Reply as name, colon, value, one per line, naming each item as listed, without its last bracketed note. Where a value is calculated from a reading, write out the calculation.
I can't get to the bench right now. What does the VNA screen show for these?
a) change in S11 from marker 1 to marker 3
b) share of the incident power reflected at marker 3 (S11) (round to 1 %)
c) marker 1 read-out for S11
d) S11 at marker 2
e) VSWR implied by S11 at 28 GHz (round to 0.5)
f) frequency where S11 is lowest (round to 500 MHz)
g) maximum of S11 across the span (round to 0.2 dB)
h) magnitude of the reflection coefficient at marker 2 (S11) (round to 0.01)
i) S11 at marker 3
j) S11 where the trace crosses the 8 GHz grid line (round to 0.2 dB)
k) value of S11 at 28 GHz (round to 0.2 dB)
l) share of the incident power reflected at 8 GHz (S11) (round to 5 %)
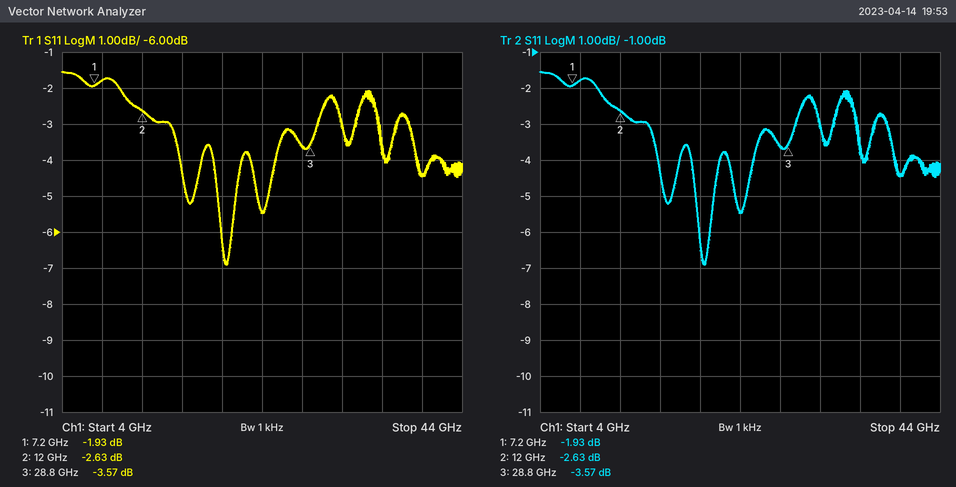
change in S11 from marker 1 to marker 3: -3.57 − (-1.93) = -1.64 dB
share of the incident power reflected at marker 3 (S11): 10^(-3.57/10) ≈ 44 %
marker 1 read-out for S11: -1.93 dB
S11 at marker 2: -2.63 dB
VSWR implied by S11 at 28 GHz: |Γ| = 10^(-3.6/20) = 0.6607; VSWR = (1 + 0.6607)/(1 − 0.6607) ≈ 4.89, so 5.0 to the nearest 0.5
frequency where S11 is lowest: 20.5 GHz
maximum of S11 across the span: -1.6 dB
magnitude of the reflection coefficient at marker 2 (S11): 10^(-2.63/20) ≈ 0.74
S11 at marker 3: -3.57 dB
S11 where the trace crosses the 8 GHz grid line: -1.8 dB
value of S11 at 28 GHz: -3.6 dB
share of the incident power reflected at 8 GHz (S11): 10^(-1.8/10) ≈ 66.1 %, so 65 % to the nearest 5 %
